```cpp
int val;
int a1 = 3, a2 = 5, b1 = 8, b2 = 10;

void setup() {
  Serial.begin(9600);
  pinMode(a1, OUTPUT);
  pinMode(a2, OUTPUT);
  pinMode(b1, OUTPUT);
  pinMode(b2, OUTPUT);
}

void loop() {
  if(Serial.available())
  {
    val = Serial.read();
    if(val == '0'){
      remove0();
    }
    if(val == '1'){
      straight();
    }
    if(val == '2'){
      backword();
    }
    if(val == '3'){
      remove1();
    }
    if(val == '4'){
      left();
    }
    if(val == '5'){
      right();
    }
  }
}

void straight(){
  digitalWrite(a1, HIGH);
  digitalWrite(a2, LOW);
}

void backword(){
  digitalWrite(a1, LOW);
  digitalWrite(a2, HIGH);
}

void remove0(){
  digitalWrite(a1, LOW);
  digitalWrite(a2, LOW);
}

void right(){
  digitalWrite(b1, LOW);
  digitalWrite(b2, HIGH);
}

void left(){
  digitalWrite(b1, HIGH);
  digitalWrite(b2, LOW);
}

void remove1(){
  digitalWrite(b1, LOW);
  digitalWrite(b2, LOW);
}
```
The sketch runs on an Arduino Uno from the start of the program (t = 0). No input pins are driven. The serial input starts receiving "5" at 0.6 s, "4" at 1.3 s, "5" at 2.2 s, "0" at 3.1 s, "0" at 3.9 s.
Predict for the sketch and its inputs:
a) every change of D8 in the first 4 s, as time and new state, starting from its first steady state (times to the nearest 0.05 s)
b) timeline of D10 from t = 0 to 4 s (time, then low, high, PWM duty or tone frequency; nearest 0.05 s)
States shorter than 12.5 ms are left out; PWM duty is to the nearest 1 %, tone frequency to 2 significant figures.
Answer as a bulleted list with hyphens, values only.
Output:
- 0 s low; 1.3 s high; 2.2 s low
- 0 s low; 0.6 s high; 1.3 s low; 2.2 s high
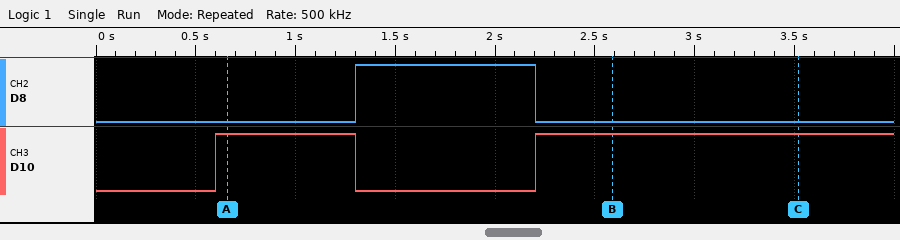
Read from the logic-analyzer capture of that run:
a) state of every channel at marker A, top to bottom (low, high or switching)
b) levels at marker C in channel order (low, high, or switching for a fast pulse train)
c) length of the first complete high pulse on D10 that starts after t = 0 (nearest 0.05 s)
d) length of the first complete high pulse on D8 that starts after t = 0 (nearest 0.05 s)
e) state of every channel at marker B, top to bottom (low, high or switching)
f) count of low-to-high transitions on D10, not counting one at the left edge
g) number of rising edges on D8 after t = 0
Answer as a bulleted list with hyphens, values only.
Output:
- D8 low, D10 high
- D8 low, D10 high
- 0.70 s
- 0.90 s
- D8 low, D10 high
- 2
- 1
